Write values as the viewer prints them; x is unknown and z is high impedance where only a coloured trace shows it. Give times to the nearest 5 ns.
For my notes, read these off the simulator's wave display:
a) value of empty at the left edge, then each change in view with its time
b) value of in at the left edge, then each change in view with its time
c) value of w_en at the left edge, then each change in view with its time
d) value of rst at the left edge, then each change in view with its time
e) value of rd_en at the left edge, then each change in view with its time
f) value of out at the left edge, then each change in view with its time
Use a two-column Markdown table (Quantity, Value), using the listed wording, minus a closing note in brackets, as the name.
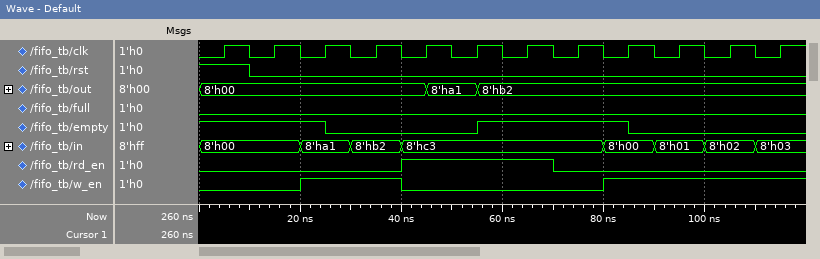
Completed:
| Quantity | Value |
|---|---|
| value of empty at the left edge, then each change in view with its time | 1, 0 at 25 ns, 1 at 55 ns, 0 at 85 ns |
| value of in at the left edge, then each change in view with its time | 8'h00, 8'ha1 at 20 ns, 8'hb2 at 30 ns, 8'hc3 at 40 ns, 8'h00 at 80 ns, 8'h01 at 90 ns, 8'h02 at 100 ns, 8'h03 at 110 ns |
| value of w_en at the left edge, then each change in view with its time | 0, 1 at 20 ns, 0 at 40 ns, 1 at 80 ns |
| value of rst at the left edge, then each change in view with its time | 1, 0 at 10 ns |
| value of rd_en at the left edge, then each change in view with its time | 0, 1 at 40 ns, 0 at 70 ns |
| value of out at the left edge, then each change in view with its time | 8'h00, 8'ha1 at 45 ns, 8'hb2 at 55 ns |
